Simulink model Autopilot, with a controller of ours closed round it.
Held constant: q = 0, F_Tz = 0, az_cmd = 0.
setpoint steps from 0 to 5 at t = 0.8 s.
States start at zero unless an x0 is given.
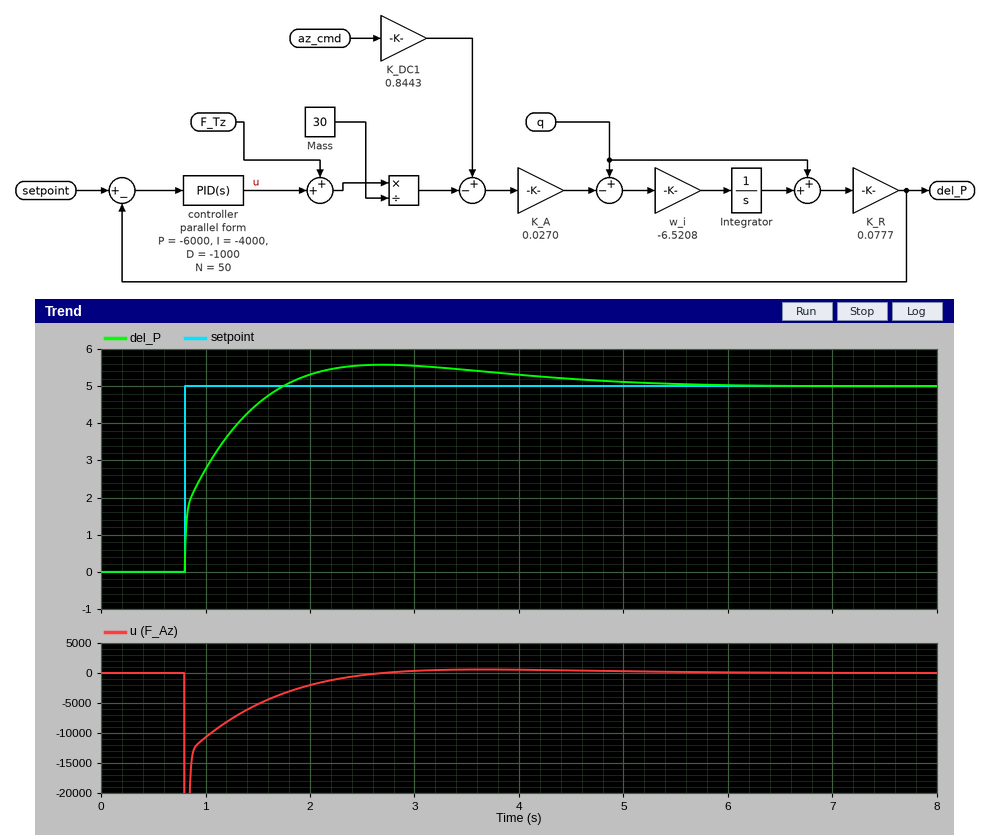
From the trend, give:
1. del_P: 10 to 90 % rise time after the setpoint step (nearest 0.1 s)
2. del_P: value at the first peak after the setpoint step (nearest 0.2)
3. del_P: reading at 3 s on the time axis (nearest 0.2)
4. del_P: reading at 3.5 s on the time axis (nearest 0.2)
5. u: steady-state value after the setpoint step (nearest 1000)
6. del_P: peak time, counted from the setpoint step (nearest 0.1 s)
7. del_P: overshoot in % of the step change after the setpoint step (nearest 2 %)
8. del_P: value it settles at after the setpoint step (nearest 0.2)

0.7 s
5.6
5.6
5.4
0
1.9 s
12 %
5.0
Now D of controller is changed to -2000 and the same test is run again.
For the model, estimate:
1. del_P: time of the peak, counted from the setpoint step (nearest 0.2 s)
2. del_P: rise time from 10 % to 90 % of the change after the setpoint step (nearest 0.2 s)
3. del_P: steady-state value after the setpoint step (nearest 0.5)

2.2 s
0.8 s
5.0
